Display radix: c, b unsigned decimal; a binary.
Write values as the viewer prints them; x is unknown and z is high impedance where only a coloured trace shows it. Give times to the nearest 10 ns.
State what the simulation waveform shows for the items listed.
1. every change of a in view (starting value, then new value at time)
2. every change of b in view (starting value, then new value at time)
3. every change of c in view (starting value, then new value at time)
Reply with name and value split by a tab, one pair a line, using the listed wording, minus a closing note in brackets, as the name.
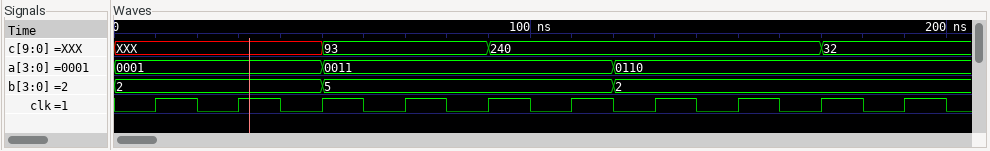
every change of a in view	0001, 0011 at 50 ns, 0110 at 120 ns
every change of b in view	2, 5 at 50 ns, 2 at 120 ns
every change of c in view	XXX, 93 at 50 ns, 240 at 90 ns, 32 at 170 ns
